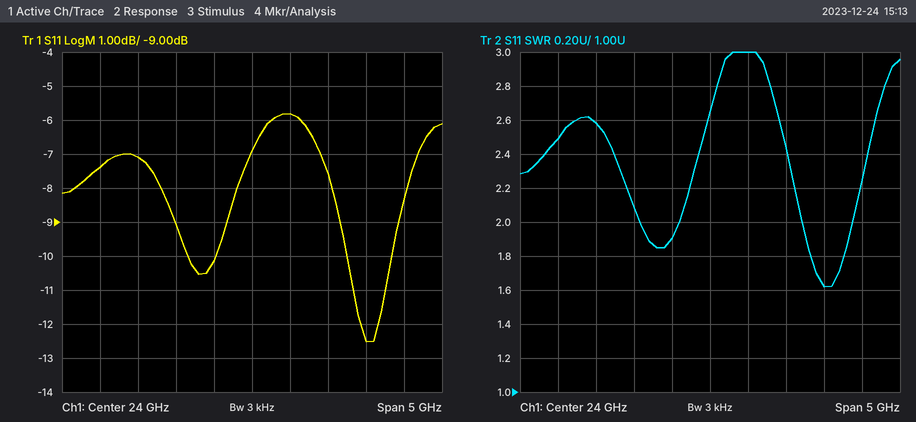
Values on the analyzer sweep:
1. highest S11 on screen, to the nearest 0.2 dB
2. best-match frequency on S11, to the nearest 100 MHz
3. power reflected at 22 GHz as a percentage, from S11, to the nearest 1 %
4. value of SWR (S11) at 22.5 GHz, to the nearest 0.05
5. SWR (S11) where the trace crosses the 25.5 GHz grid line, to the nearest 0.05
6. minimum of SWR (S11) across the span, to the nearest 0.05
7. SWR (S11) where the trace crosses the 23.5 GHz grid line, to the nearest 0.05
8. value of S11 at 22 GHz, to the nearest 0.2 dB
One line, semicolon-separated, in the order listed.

-5.8 dB; 25.5 GHz; 18 %; 2.60; 1.60; 1.60; 1.90; -7.4 dB
